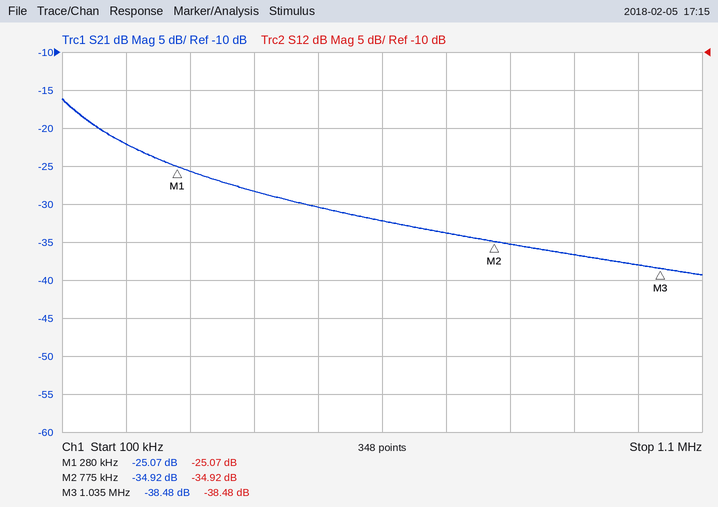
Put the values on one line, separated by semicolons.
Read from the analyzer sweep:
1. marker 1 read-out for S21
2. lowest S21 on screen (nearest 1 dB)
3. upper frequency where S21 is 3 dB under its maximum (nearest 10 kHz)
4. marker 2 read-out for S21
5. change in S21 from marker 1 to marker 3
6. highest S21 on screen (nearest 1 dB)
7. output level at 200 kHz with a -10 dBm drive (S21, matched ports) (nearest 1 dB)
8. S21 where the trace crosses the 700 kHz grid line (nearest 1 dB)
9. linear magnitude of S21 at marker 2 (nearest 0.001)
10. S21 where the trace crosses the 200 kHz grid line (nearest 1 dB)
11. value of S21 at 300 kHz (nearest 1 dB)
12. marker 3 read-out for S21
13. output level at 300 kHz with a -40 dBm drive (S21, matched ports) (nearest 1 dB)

-25.07 dB; -39 dB; 140 kHz; -34.92 dB; -13.41 dB; -16 dB; -32 dBm; -34 dB; 0.018; -22 dB; -26 dB; -38.48 dB; -66 dBm
